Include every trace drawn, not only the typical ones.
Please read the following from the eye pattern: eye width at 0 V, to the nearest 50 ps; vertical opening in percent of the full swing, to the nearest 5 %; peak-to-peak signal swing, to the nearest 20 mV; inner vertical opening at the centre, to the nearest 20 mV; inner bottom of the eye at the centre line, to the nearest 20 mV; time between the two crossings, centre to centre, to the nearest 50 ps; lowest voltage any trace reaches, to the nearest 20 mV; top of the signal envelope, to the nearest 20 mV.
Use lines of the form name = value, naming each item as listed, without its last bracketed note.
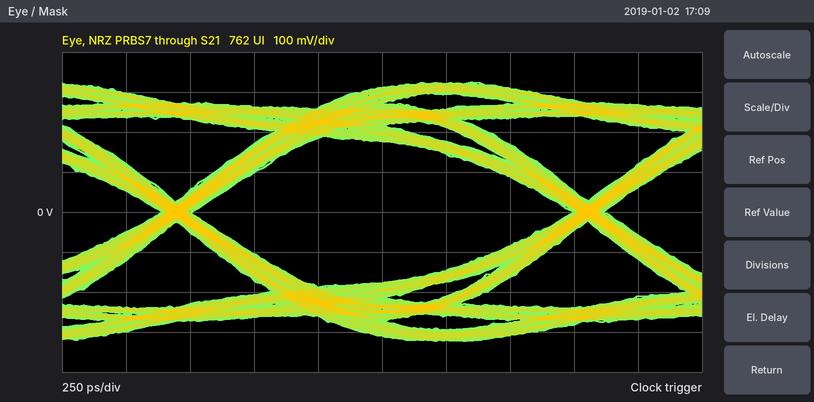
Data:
eye width at 0 V, to the nearest 50 ps = 1.50 ns
vertical opening in percent of the full swing, to the nearest 5 % = 55 %
peak-to-peak signal swing, to the nearest 20 mV = 640 mV
inner vertical opening at the centre, to the nearest 20 mV = 360 mV
inner bottom of the eye at the centre line, to the nearest 20 mV = -180 mV
time between the two crossings, centre to centre, to the nearest 50 ps = 1.60 ns
lowest voltage any trace reaches, to the nearest 20 mV = -320 mV
top of the signal envelope, to the nearest 20 mV = 320 mV
